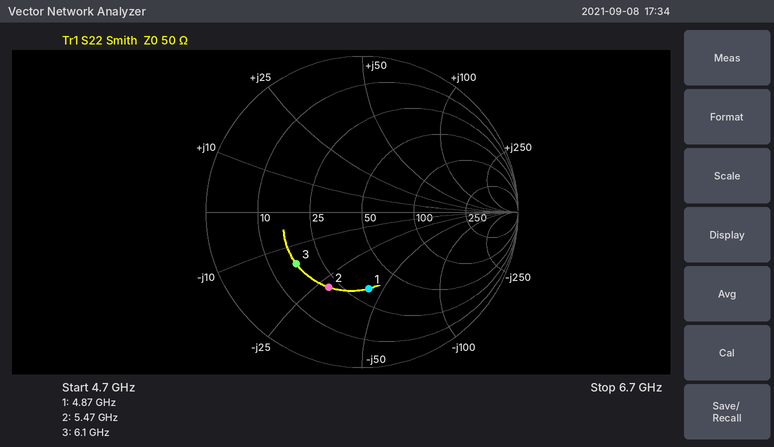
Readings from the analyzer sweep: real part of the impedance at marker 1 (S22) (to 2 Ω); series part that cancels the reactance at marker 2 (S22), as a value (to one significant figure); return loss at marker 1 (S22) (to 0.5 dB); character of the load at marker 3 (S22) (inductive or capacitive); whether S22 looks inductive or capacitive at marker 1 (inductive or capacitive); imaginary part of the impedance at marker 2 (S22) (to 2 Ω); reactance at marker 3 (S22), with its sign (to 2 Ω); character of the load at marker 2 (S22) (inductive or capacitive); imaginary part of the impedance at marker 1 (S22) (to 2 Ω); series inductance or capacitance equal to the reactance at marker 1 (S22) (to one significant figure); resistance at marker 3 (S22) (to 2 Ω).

32 Ω
800 pH
6.0 dB
capacitive
capacitive
-28 Ω
-16 Ω
capacitive
-42 Ω
800 fF
16 Ω
